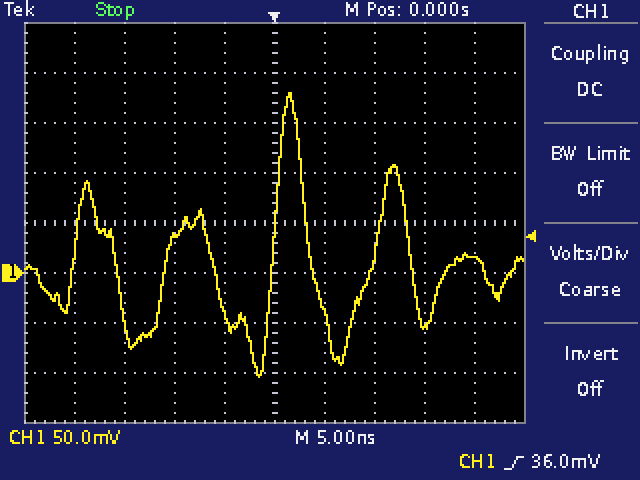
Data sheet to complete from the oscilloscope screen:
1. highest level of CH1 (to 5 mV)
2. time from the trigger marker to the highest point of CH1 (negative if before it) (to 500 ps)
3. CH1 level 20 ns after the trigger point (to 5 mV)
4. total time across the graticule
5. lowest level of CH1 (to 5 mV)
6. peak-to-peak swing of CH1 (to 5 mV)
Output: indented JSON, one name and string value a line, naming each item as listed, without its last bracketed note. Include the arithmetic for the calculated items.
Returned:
{
  "highest level of CH1": "180 mV",
  "time from the trigger marker to the highest point of CH1 (negative if before it)": "+1.5 ns",
  "CH1 level 20 ns after the trigger point": "15 mV",
  "total time across the graticule": "50 ns",
  "lowest level of CH1": "-105 mV",
  "peak-to-peak swing of CH1": "180 mV − (-105 mV) = 285 mV"
}
